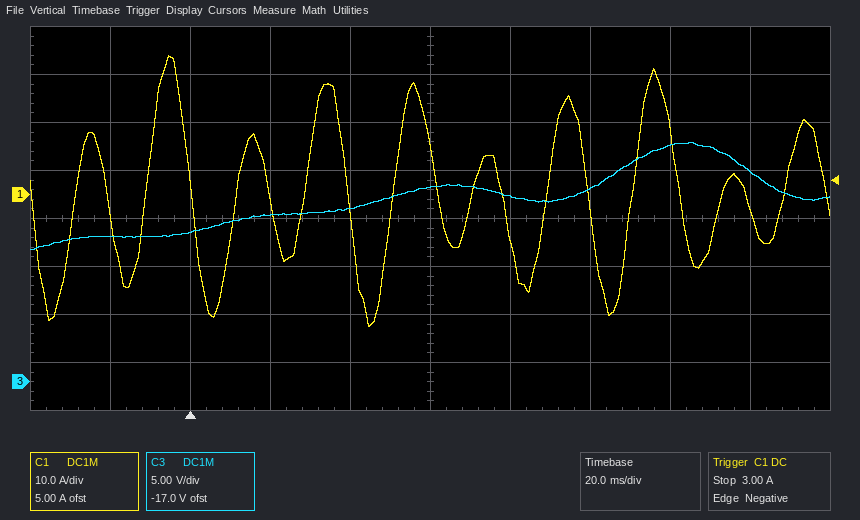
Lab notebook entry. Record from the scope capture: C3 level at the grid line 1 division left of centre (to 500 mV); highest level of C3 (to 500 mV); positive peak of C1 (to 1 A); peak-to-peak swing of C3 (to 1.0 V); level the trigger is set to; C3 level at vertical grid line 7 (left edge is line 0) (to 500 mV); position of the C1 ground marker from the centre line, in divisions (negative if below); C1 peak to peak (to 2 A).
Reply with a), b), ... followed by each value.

a) 18.0 V
b) 25.0 V
c) 29 A
d) 11.0 V
e) 3.00 A
f) 20.0 V
g) +0.5 div
h) 56 A
